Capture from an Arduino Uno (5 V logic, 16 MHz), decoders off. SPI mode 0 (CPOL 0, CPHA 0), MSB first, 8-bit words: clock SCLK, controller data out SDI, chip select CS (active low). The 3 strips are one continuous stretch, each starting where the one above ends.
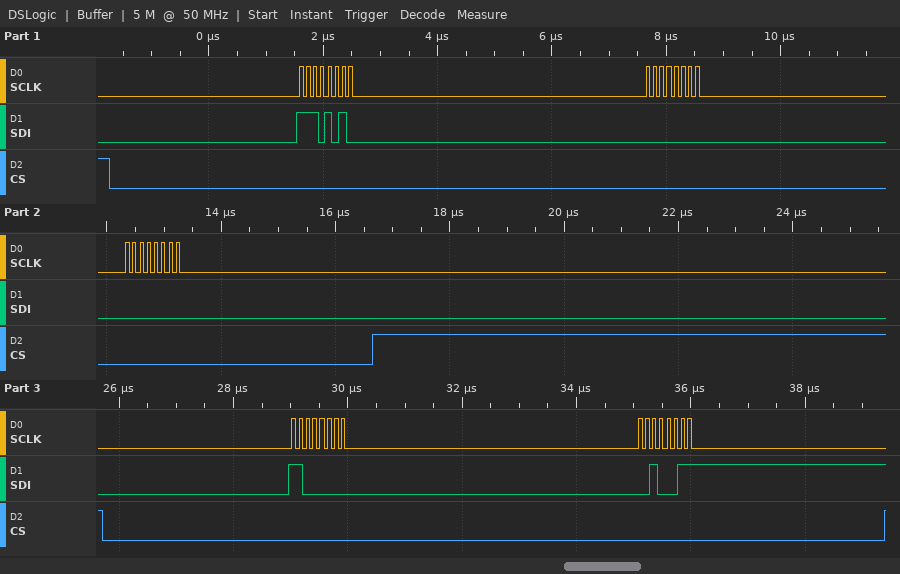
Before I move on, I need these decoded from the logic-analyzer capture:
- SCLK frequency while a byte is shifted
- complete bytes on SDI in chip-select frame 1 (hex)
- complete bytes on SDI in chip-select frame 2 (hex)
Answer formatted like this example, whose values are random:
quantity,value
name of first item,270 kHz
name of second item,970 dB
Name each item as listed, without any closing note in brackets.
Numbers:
quantity,value
SCLK frequency while a byte is shifted,8 MHz
complete bytes on SDI in chip-select frame 1,EA 00 00
complete bytes on SDI in chip-select frame 2,C0 23
